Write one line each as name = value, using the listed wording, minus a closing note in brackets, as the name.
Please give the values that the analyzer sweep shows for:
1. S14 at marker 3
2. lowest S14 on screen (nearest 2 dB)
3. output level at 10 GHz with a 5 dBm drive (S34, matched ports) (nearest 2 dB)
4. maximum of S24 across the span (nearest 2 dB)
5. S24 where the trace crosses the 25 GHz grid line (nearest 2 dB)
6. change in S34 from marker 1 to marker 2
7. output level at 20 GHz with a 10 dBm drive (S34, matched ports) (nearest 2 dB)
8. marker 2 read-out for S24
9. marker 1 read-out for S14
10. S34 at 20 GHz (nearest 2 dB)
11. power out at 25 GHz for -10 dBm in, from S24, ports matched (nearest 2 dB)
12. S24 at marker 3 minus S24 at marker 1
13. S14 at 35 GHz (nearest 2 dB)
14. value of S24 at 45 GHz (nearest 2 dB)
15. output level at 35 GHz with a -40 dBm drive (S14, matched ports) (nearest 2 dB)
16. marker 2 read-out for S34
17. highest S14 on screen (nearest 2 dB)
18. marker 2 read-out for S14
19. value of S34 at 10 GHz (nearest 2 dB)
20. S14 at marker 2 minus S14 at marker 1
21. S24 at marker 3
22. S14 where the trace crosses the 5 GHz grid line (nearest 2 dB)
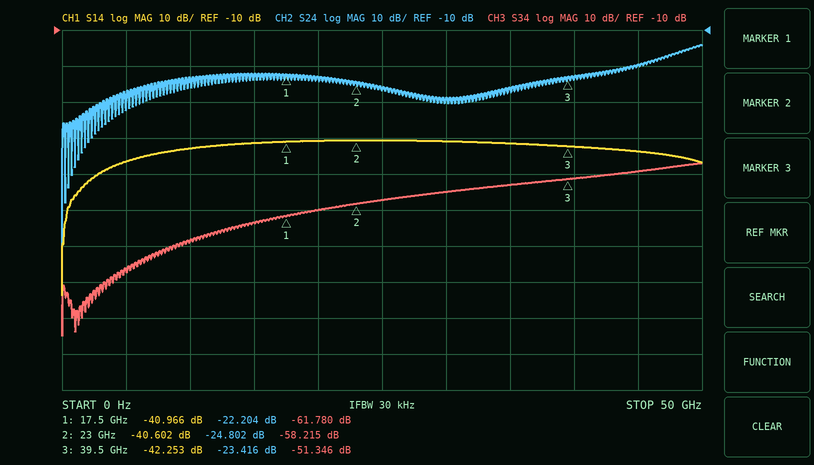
S14 at marker 3 = -42.253 dB
lowest S14 on screen = -84 dB
output level at 10 GHz with a 5 dBm drive (S34, matched ports) = -64 dBm
maximum of S24 across the span = -14 dB
S24 where the trace crosses the 25 GHz grid line = -26 dB
change in S34 from marker 1 to marker 2 = 3.565 dB
output level at 20 GHz with a 10 dBm drive (S34, matched ports) = -50 dBm
marker 2 read-out for S24 = -24.802 dB
marker 1 read-out for S14 = -40.966 dB
S34 at 20 GHz = -60 dB
power out at 25 GHz for -10 dBm in, from S24, ports matched = -36 dBm
S24 at marker 3 minus S24 at marker 1 = -1.212 dB
S14 at 35 GHz = -42 dB
value of S24 at 45 GHz = -20 dB
output level at 35 GHz with a -40 dBm drive (S14, matched ports) = -82 dBm
marker 2 read-out for S34 = -58.215 dB
highest S14 on screen = -40 dB
marker 2 read-out for S14 = -40.602 dB
value of S34 at 10 GHz = -68 dB
S14 at marker 2 minus S14 at marker 1 = 0.364 dB
S24 at marker 3 = -23.416 dB
S14 where the trace crosses the 5 GHz grid line = -46 dB
